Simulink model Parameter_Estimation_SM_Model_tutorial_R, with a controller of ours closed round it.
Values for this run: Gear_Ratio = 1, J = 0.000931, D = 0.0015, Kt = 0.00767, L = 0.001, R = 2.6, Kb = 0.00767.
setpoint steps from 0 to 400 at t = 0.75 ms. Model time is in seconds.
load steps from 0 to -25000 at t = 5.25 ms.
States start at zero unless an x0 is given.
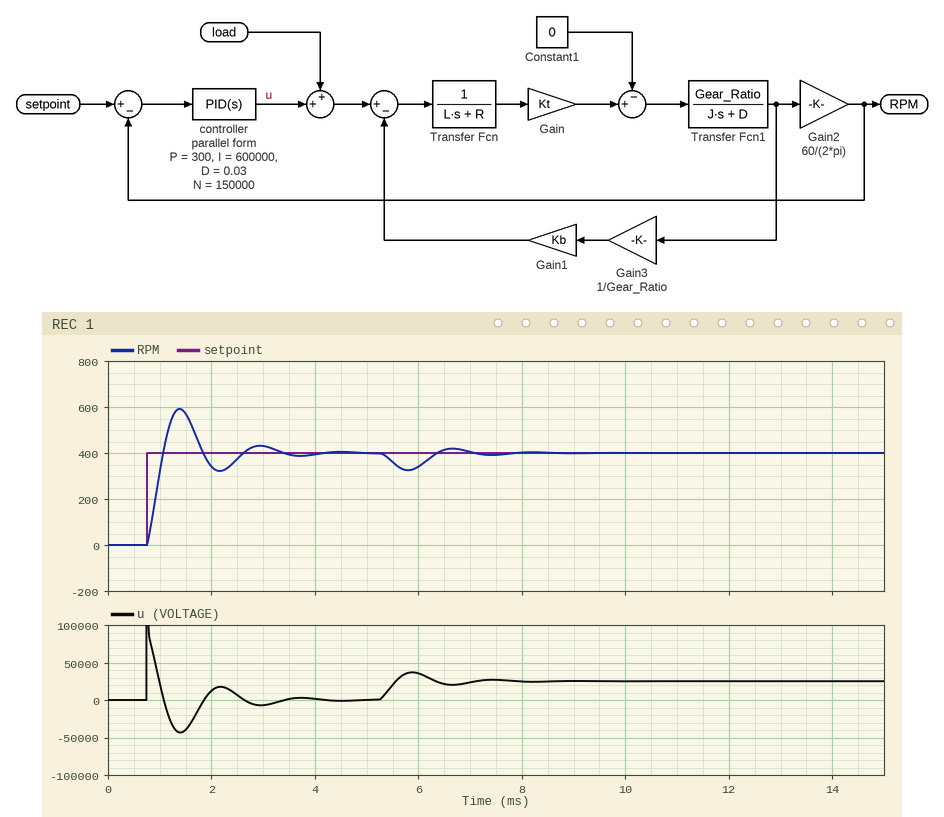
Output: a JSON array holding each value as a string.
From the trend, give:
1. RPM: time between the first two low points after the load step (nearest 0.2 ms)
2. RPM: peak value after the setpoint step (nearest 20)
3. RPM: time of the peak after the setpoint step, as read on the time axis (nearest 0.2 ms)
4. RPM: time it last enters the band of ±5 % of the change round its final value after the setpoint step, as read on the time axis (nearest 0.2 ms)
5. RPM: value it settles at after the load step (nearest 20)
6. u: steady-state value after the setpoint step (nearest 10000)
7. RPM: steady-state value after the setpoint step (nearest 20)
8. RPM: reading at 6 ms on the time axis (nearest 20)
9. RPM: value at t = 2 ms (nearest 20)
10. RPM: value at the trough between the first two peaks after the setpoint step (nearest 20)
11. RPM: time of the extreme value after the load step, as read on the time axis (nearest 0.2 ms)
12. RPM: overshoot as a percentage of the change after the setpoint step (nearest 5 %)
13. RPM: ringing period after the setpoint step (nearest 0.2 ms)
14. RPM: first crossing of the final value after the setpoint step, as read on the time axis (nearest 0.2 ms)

["1.6 ms", "600", "1.4 ms", "3.2 ms", "400", "0", "400", "340", "340", "320", "5.8 ms", "50 %", "1.6 ms", "1.0 ms"]
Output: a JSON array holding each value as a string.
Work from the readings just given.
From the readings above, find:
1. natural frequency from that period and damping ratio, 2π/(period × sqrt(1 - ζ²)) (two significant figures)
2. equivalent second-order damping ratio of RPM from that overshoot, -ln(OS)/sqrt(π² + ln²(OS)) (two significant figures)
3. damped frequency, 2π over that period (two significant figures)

["4.0 rad/ms", "0.22", "3.9 rad/ms"]
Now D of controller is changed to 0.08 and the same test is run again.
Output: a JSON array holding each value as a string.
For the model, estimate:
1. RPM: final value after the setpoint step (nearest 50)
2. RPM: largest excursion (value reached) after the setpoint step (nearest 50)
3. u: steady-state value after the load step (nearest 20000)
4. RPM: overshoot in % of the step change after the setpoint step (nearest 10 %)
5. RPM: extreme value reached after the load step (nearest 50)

["400", "500", "20000", "20 %", "350"]
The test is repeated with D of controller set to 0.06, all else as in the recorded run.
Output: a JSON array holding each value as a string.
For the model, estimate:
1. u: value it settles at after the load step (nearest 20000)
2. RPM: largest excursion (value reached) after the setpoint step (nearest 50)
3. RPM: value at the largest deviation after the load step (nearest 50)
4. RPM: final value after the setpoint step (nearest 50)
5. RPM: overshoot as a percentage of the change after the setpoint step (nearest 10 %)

["20000", "500", "350", "400", "30 %"]
